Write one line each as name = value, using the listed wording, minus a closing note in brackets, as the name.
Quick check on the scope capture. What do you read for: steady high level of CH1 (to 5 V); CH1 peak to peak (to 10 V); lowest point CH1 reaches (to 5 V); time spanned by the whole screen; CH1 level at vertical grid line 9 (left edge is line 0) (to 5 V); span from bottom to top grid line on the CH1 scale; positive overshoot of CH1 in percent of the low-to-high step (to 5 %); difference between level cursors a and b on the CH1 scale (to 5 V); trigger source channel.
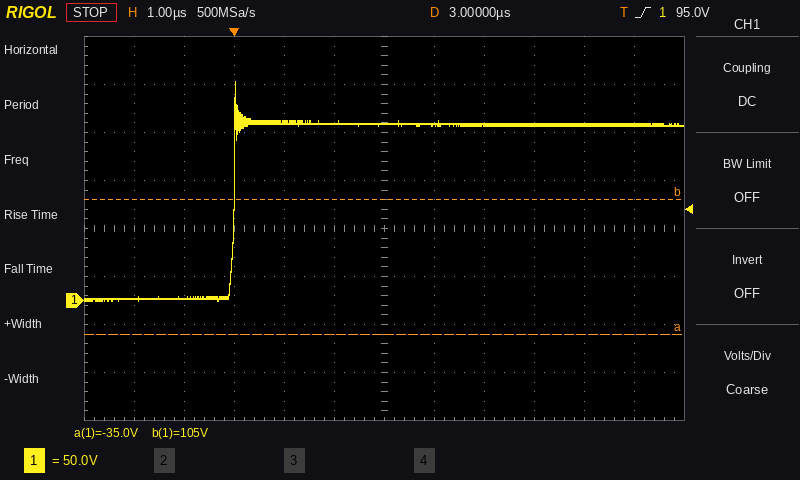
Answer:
steady high level of CH1 = 185 V
CH1 peak to peak = 230 V
lowest point CH1 reaches = 0 V
time spanned by the whole screen = 12 µs
CH1 level at vertical grid line 9 (left edge is line 0) = 185 V
span from bottom to top grid line on the CH1 scale = 400 V
positive overshoot of CH1 in percent of the low-to-high step = 25 %
difference between level cursors a and b on the CH1 scale = 140 V
trigger source channel = CH1
